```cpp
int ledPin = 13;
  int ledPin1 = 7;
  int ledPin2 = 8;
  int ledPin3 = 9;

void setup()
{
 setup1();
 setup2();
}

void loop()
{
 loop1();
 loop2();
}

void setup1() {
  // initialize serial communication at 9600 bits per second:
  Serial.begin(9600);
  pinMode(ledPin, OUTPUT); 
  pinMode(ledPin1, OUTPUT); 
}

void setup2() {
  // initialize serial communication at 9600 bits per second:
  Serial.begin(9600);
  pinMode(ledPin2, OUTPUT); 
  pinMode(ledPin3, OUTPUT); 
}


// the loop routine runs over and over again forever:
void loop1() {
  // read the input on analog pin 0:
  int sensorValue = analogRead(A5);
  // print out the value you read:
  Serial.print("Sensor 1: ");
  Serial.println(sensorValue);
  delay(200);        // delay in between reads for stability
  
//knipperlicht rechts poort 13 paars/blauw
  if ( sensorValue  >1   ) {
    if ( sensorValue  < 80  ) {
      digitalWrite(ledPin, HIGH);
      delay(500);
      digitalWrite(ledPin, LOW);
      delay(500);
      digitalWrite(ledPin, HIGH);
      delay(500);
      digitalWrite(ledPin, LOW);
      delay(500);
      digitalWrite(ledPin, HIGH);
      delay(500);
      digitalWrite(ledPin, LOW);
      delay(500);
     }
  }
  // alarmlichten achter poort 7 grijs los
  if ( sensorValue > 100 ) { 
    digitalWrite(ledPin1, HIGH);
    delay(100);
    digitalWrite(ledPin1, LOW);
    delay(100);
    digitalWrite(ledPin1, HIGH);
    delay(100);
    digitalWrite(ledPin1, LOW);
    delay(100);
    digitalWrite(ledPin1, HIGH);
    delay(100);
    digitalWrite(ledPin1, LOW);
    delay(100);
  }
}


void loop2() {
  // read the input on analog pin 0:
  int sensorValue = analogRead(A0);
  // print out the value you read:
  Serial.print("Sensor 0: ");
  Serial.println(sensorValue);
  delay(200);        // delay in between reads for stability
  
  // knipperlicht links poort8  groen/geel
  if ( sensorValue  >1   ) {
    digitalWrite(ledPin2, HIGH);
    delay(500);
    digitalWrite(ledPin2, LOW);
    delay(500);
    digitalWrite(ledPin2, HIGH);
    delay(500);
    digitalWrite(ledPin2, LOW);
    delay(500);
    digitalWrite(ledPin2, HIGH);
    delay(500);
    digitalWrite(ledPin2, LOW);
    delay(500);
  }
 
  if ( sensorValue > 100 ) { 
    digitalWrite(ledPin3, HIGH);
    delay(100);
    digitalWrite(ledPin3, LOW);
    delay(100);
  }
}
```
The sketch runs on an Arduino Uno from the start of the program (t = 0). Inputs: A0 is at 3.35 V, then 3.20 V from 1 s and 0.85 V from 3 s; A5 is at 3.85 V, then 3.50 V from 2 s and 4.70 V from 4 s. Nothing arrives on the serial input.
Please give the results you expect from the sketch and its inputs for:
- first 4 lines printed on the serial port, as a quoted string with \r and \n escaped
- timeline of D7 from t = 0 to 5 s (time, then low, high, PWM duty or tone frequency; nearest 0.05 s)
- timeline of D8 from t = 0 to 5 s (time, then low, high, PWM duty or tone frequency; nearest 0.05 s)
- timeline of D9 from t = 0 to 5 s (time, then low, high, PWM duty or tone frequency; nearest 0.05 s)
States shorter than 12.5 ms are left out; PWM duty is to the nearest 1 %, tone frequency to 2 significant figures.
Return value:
"Sensor 1: 788\r\nSensor 0: 686\r\nSensor 1: 962\r\nSensor 0: 174\r\n"
0 s low; 0.2 s high; 0.3 s low; 0.4 s high; 0.5 s low; 0.6 s high; 0.7 s low; 4.4 s high; 4.5 s low; 4.6 s high; 4.7 s low; 4.8 s high; 4.9 s low
0 s low; 1 s high; 1.5 s low; 2 s high; 2.5 s low; 3 s high; 3.5 s low
0 s low; 4 s high; 4.1 s low
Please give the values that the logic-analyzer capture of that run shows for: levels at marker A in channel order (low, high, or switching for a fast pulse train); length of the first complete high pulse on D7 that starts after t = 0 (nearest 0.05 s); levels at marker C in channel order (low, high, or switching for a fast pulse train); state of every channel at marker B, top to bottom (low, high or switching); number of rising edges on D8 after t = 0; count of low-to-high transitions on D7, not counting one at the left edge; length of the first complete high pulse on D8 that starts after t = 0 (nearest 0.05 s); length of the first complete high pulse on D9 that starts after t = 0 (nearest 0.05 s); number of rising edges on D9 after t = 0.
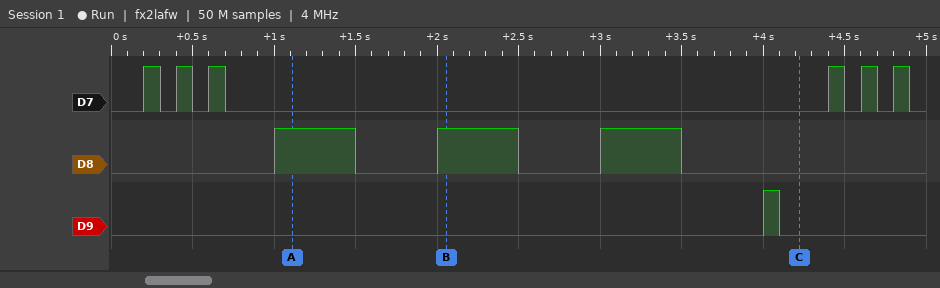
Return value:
D7 low, D8 high, D9 low
0.10 s
D7 low, D8 low, D9 low
D7 low, D8 high, D9 low
3
6
0.50 s
0.10 s
1
